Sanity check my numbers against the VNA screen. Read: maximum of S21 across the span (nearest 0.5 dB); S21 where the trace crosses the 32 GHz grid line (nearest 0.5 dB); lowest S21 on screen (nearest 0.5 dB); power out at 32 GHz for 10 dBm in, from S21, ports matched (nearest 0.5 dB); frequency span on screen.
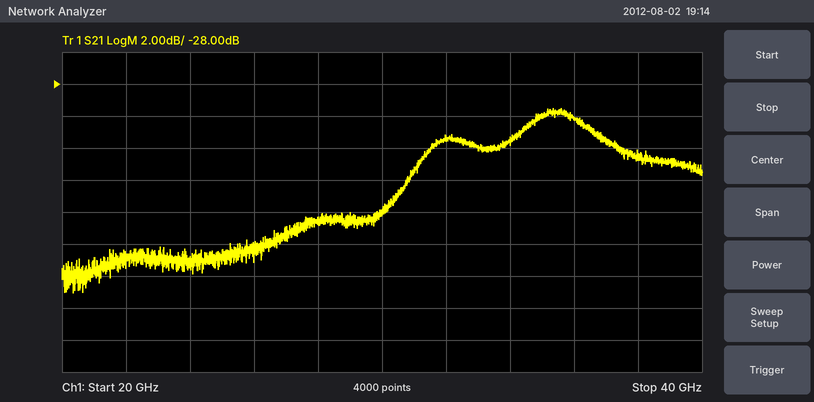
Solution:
-29.5 dB
-31.5 dB
-41.0 dB
-21.5 dBm
20 GHz
